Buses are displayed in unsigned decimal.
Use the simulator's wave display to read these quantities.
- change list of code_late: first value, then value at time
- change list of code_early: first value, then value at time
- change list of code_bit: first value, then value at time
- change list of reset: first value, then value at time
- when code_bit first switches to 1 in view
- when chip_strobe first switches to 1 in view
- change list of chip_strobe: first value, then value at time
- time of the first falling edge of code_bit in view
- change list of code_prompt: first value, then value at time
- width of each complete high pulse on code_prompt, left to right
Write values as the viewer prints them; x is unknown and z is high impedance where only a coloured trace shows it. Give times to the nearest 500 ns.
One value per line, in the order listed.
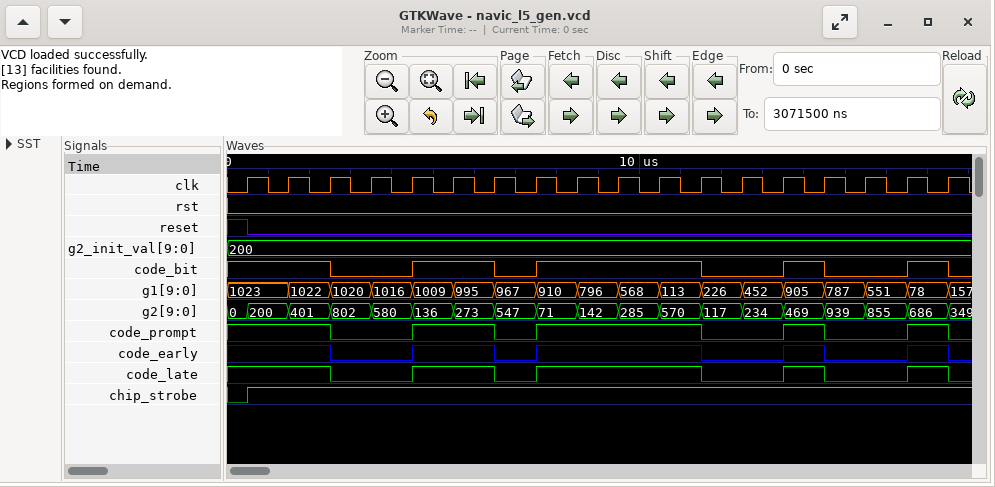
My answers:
1, 0 at 2500 ns, 1 at 4500 ns, 0 at 6500 ns, 1 at 7500 ns, 0 at 11500 ns, 1 at 13500 ns, 0 at 14500 ns, 1 at 16500 ns, 0 at 17500 ns
1, 0 at 2500 ns, 1 at 4500 ns, 0 at 6500 ns, 1 at 7500 ns, 0 at 11500 ns, 1 at 13500 ns, 0 at 14500 ns, 1 at 16500 ns, 0 at 17500 ns
1, 0 at 2500 ns, 1 at 4500 ns, 0 at 6500 ns, 1 at 7500 ns, 0 at 11500 ns, 1 at 13500 ns, 0 at 14500 ns, 1 at 16500 ns, 0 at 17500 ns
1, 0 at 500 ns
4500 ns
500 ns
0, 1 at 500 ns
2500 ns
1, 0 at 2500 ns, 1 at 4500 ns, 0 at 6500 ns, 1 at 7500 ns, 0 at 11500 ns, 1 at 13500 ns, 0 at 14500 ns, 1 at 16500 ns, 0 at 17500 ns
2000 ns, 4000 ns, 1000 ns, 1000 ns
